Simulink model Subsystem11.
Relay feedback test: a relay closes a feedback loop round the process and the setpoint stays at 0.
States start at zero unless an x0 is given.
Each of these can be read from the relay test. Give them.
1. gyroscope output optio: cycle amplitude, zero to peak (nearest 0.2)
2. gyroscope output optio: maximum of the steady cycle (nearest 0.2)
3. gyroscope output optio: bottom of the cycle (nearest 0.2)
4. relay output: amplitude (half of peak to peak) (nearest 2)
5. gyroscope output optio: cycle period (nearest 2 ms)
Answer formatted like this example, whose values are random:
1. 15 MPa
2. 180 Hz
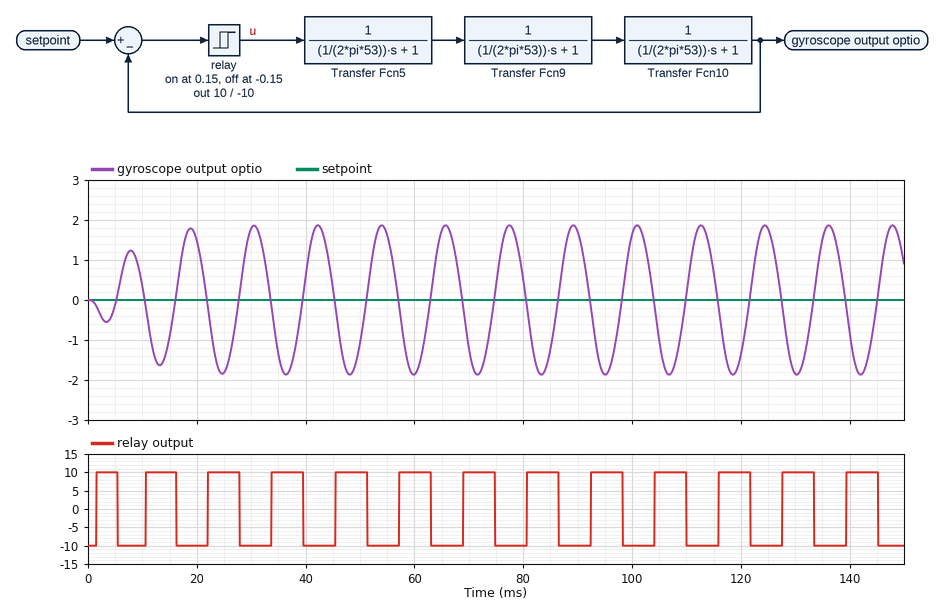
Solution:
1. 1.8
2. 1.8
3. -1.8
4. 10
5. 12 ms
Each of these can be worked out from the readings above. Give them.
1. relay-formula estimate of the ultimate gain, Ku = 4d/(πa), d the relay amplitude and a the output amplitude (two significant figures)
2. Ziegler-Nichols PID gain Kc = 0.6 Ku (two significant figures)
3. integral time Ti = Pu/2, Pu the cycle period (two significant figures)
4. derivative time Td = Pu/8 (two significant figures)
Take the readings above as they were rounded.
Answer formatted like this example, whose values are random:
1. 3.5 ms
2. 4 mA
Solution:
1. 7.1
2. 4.3
3. 6.0 ms
4. 1.5 ms
